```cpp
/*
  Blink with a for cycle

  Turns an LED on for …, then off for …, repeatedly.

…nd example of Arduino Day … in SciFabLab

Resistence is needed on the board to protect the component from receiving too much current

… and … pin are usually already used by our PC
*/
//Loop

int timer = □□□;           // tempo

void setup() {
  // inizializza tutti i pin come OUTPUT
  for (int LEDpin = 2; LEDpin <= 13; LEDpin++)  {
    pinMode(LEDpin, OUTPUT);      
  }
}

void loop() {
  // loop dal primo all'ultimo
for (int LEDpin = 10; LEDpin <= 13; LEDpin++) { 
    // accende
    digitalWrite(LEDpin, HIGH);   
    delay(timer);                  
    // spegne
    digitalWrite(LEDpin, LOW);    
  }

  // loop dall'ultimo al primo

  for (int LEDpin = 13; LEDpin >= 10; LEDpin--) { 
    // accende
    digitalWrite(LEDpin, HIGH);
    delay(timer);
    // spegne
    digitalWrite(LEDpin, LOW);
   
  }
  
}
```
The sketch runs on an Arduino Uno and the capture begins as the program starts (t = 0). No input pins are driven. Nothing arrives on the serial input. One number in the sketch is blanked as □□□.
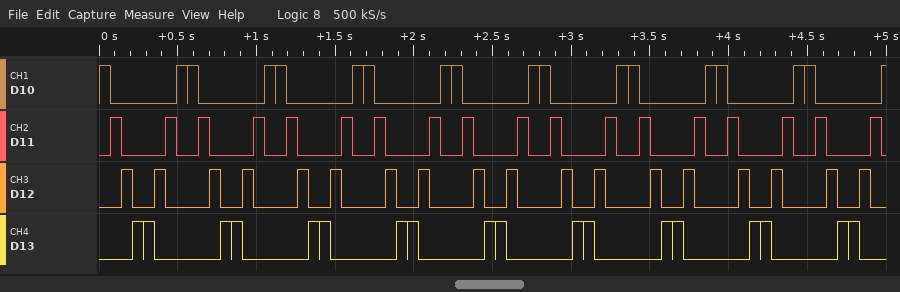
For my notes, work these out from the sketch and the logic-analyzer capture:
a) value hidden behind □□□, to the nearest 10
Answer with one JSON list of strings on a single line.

["70"]
